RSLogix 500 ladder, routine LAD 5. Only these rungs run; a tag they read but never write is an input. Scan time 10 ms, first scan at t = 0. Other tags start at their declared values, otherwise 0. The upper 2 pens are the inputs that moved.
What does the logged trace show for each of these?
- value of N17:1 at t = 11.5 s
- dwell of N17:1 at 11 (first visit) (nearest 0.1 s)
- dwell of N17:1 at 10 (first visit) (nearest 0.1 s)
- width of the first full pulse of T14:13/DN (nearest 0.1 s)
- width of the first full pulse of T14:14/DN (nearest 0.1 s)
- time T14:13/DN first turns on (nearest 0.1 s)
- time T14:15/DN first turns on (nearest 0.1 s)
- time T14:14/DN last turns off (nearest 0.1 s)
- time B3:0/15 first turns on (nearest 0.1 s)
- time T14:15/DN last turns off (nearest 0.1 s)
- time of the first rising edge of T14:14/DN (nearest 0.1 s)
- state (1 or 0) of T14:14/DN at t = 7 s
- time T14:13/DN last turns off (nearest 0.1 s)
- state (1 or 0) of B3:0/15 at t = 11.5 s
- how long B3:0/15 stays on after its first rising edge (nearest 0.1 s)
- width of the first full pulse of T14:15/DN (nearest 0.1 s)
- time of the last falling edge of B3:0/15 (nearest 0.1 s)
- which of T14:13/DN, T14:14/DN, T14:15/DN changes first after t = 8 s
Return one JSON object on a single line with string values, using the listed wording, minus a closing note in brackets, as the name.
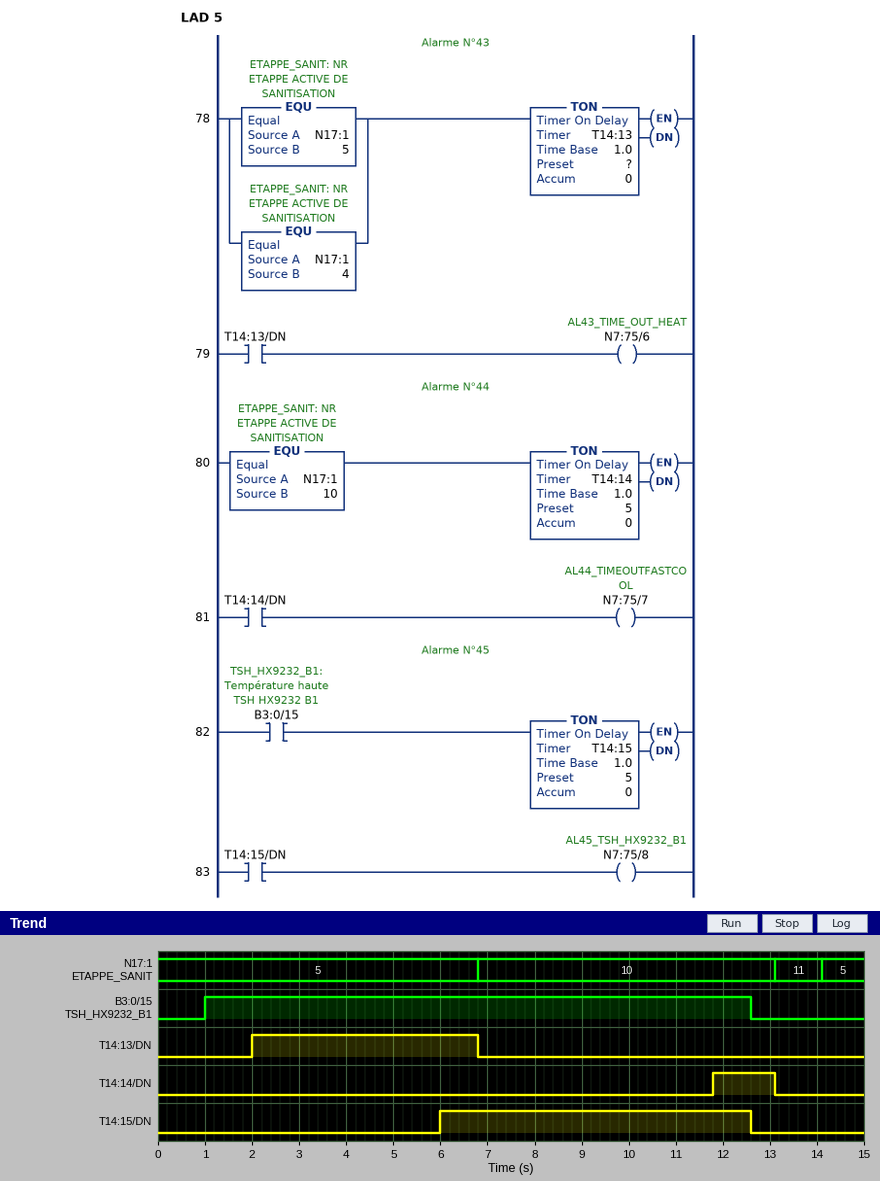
{"value of N17:1 at t = 11.5 s": "10", "dwell of N17:1 at 11 (first visit)": "1.0 s", "dwell of N17:1 at 10 (first visit)": "6.3 s", "width of the first full pulse of T14:13/DN": "4.8 s", "width of the first full pulse of T14:14/DN": "1.3 s", "time T14:13/DN first turns on": "2.0 s", "time T14:15/DN first turns on": "6.0 s", "time T14:14/DN last turns off": "13.1 s", "time B3:0/15 first turns on": "1.0 s", "time T14:15/DN last turns off": "12.6 s", "time of the first rising edge of T14:14/DN": "11.8 s", "state (1 or 0) of T14:14/DN at t = 7 s": "0", "time T14:13/DN last turns off": "6.8 s", "state (1 or 0) of B3:0/15 at t = 11.5 s": "1", "how long B3:0/15 stays on after its first rising edge": "11.6 s", "width of the first full pulse of T14:15/DN": "6.6 s", "time of the last falling edge of B3:0/15": "12.6 s", "which of T14:13/DN, T14:14/DN, T14:15/DN changes first after t = 8 s": "T14:14/DN"}
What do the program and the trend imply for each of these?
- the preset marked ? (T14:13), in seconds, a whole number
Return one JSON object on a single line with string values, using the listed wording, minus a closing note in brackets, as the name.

{"the preset marked ? (T14:13), in seconds, a whole number": "2 s"}
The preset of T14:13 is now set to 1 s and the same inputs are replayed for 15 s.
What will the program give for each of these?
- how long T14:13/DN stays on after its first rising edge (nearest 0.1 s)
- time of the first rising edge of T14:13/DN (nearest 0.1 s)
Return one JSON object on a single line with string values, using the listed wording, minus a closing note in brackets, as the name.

{"how long T14:13/DN stays on after its first rising edge": "5.8 s", "time of the first rising edge of T14:13/DN": "1.0 s"}
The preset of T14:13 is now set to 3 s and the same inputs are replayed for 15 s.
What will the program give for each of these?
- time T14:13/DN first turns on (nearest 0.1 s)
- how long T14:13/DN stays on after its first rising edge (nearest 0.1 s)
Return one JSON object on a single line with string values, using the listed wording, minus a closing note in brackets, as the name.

{"time T14:13/DN first turns on": "3.0 s", "how long T14:13/DN stays on after its first rising edge": "3.8 s"}
